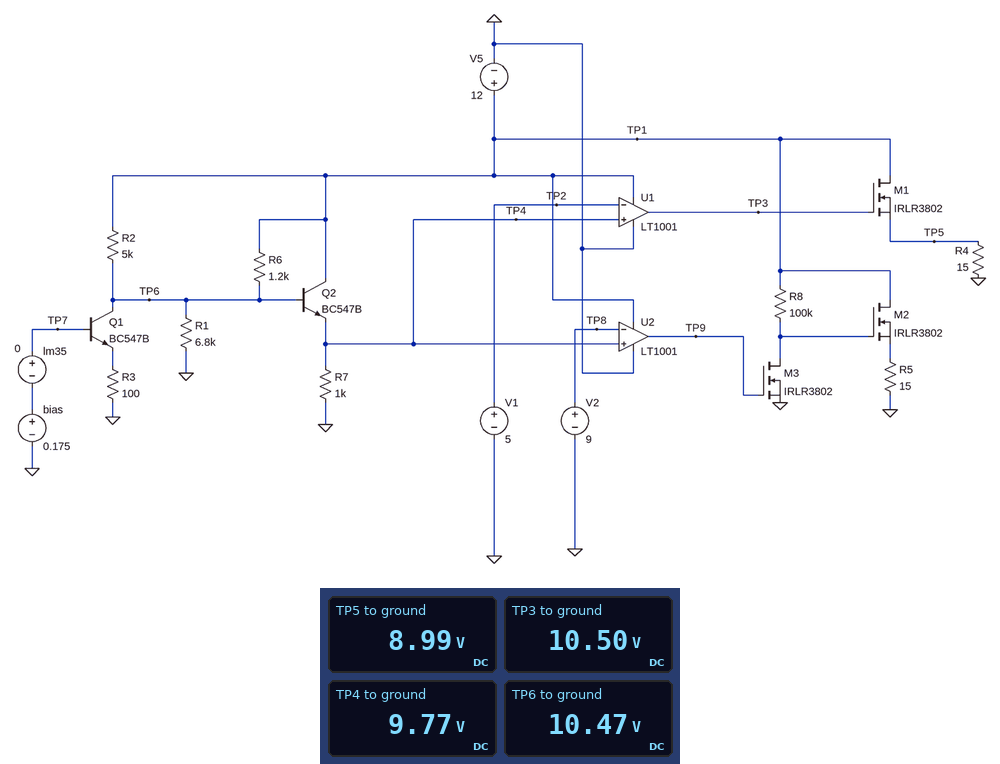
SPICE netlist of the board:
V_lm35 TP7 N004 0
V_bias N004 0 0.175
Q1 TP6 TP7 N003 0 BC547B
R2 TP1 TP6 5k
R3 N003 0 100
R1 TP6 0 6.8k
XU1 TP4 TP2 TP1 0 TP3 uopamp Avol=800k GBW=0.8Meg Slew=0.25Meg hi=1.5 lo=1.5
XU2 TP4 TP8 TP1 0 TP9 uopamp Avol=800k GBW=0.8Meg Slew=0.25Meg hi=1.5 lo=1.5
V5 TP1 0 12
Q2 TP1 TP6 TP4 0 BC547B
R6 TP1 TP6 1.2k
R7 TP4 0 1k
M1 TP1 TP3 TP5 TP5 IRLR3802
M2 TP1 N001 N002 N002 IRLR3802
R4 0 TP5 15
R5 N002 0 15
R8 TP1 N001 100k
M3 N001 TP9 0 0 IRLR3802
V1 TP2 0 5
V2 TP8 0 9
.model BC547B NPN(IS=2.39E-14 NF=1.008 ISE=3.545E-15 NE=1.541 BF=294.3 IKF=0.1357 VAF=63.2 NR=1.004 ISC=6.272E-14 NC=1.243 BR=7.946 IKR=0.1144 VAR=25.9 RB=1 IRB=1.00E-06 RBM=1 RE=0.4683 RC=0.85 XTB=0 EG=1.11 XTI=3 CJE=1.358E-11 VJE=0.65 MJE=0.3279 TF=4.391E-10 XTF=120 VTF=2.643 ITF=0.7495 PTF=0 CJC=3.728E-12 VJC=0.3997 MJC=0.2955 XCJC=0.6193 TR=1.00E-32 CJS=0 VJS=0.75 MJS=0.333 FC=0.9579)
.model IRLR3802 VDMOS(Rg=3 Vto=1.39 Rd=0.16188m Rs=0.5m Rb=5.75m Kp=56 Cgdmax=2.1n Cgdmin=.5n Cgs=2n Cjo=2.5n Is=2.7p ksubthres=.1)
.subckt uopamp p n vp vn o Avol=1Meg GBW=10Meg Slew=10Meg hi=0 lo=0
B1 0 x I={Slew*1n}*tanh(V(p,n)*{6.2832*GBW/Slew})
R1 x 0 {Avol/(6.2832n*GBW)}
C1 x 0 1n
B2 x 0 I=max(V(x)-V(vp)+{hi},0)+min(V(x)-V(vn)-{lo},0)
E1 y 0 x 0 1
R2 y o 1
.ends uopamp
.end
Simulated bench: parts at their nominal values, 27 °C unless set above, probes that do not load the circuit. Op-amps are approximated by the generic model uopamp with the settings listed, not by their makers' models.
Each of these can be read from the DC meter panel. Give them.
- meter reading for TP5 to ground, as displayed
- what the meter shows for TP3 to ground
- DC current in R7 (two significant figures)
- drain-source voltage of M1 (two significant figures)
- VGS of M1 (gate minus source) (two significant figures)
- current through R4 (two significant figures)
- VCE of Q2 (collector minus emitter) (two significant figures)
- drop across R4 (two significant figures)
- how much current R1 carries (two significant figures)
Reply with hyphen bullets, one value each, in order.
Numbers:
- 8.99 V
- 10.50 V
- 9.8 mA
- 3.0 V
- 1.5 V
- 600 mA
- 2.2 V
- 9.0 V
- 1.5 mA
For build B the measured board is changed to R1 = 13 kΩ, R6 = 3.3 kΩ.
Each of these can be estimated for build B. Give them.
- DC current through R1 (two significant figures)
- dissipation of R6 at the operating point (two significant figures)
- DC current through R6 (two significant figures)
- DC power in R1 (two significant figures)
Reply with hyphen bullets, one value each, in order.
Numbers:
- 800 µA
- 830 µW
- 500 µA
- 8.2 mW
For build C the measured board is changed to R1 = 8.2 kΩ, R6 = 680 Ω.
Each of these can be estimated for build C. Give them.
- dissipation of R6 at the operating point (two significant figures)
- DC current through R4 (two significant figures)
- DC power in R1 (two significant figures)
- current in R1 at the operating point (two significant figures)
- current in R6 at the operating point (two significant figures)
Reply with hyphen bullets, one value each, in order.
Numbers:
- 1.0 mW
- 600 mA
- 15 mW
- 1.4 mA
- 1.2 mA
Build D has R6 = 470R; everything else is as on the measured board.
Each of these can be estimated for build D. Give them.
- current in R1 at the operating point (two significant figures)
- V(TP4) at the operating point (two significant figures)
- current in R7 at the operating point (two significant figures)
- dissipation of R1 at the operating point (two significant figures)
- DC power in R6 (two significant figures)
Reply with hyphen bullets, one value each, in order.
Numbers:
- 1.7 mA
- 11 V
- 11 mA
- 19 mW
- 1.1 mW
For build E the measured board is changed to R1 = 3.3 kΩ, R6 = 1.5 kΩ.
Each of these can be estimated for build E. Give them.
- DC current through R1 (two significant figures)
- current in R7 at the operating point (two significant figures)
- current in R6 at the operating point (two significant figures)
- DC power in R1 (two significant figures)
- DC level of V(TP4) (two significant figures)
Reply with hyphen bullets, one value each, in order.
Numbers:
- 2.7 mA
- 8.2 mA
- 2.1 mA
- 24 mW
- 8.2 V
